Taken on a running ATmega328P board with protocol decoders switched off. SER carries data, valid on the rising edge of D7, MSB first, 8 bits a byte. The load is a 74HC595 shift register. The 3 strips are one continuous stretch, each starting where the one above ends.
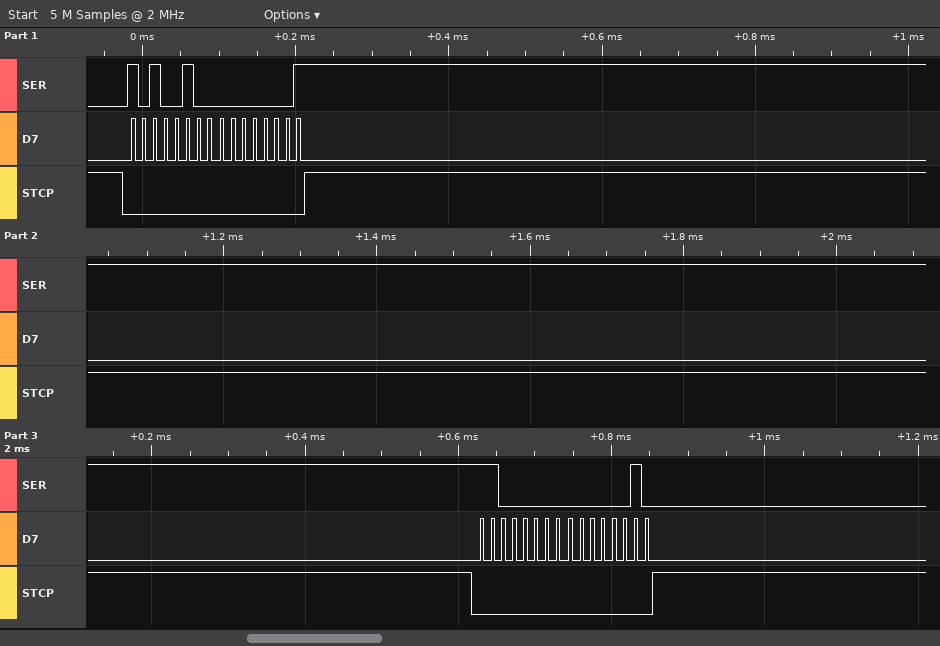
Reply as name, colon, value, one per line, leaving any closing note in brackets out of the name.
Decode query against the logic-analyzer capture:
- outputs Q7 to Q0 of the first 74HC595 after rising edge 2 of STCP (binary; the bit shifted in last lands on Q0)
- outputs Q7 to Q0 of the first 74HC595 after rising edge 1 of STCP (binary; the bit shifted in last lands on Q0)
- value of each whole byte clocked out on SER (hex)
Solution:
outputs Q7 to Q0 of the first 74HC595 after rising edge 2 of STCP: 00000010
outputs Q7 to Q0 of the first 74HC595 after rising edge 1 of STCP: 00000001
value of each whole byte clocked out on SER: A4 01 C0 02
